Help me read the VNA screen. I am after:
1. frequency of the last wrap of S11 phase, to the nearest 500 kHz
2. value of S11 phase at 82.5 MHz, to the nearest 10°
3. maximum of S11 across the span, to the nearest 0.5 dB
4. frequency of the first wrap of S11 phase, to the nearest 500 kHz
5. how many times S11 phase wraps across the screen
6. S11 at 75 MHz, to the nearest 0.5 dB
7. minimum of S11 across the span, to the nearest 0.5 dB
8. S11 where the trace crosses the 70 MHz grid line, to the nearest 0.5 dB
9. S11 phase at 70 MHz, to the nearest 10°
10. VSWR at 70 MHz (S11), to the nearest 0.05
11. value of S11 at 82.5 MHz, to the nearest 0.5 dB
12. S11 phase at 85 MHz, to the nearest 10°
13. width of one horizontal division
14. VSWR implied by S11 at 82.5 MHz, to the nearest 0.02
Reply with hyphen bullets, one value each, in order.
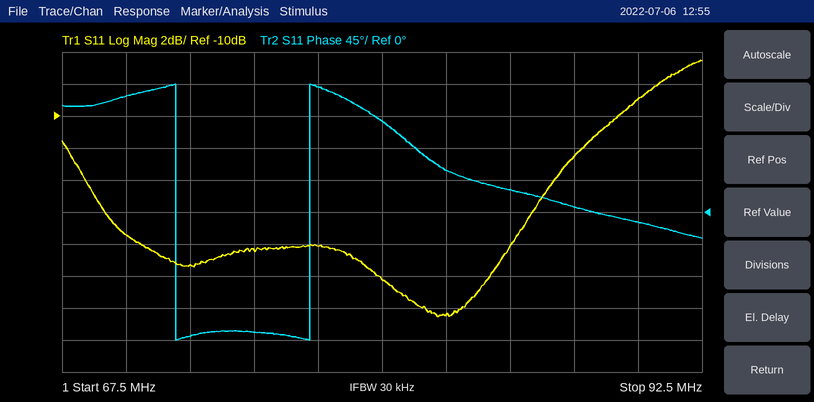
- 77.0 MHz
- 60°
- -6.5 dB
- 72.0 MHz
- 2
- -18.5 dB
- -22.5 dB
- -17.5 dB
- 160°
- 1.30
- -22.5 dB
- 30°
- 2.5 MHz
- 1.16
